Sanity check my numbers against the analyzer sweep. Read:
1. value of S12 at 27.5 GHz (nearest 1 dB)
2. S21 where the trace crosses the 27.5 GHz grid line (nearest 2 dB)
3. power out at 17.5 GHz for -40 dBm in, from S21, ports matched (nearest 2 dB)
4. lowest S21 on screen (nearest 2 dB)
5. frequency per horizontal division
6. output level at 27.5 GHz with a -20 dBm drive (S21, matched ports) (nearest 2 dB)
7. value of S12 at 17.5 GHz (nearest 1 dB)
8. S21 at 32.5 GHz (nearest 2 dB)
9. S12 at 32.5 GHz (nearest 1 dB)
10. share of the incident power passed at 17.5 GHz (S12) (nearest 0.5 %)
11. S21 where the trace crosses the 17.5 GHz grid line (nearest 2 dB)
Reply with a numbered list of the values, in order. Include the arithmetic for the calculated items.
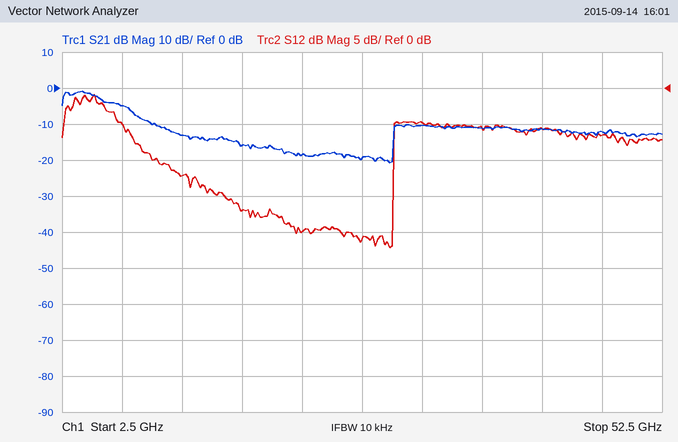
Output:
1. -21 dB
2. -20 dB
3. -40 dBm + (-16 dB) = -56 dBm
4. -20 dB
5. 5 GHz
6. -20 dBm + (-20 dB) = -40 dBm
7. -17 dB
8. -10 dB
9. -5 dB
10. 10^(-17/10) ≈ 2.0 %
11. -16 dB
